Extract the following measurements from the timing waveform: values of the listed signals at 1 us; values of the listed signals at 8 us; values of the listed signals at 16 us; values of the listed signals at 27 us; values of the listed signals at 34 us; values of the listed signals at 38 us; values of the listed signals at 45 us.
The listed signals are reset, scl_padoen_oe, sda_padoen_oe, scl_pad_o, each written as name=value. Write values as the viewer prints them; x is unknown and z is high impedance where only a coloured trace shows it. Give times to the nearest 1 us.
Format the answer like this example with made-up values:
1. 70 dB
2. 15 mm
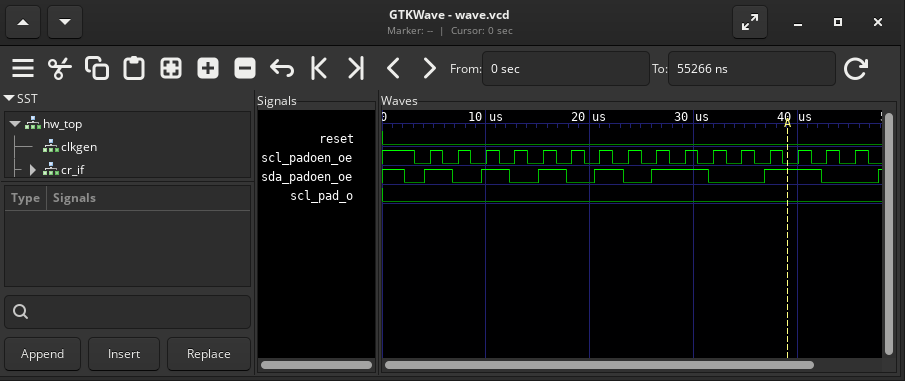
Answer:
1. reset=0, scl_padoen_oe=1, sda_padoen_oe=1, scl_pad_o=0
2. reset=0, scl_padoen_oe=1, sda_padoen_oe=0, scl_pad_o=0
3. reset=0, scl_padoen_oe=1, sda_padoen_oe=1, scl_pad_o=0
4. reset=0, scl_padoen_oe=1, sda_padoen_oe=1, scl_pad_o=0
5. reset=0, scl_padoen_oe=0, sda_padoen_oe=0, scl_pad_o=0
6. reset=0, scl_padoen_oe=1, sda_padoen_oe=1, scl_pad_o=0
7. reset=0, scl_padoen_oe=0, sda_padoen_oe=0, scl_pad_o=0
